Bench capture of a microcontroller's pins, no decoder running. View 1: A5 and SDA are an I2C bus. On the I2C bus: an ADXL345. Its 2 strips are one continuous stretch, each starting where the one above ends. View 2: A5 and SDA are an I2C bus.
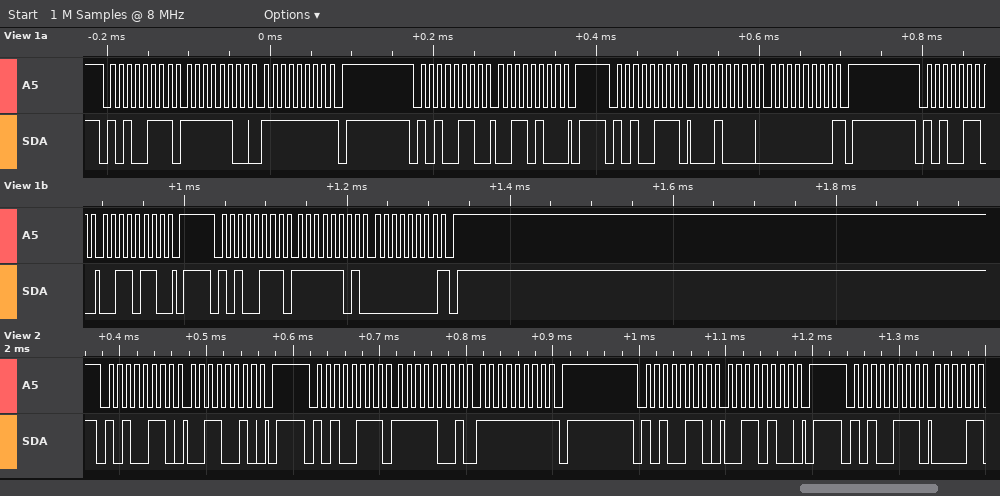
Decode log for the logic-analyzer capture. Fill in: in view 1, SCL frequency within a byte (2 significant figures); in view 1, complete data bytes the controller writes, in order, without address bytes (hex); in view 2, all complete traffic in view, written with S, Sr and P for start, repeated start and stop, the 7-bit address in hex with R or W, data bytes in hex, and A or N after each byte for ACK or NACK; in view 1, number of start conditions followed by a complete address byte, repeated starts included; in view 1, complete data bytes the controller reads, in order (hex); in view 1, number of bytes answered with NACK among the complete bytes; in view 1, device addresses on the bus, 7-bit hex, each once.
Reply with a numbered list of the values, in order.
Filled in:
1. 100 kHz
2. 34 36
3. S 53W A 32 A P S 53R A F9 A FF N P S 53W A 34 A P S 53R A
4. 5
5. FC FF 10 00 FD 00
6. 3
7. 0x53
